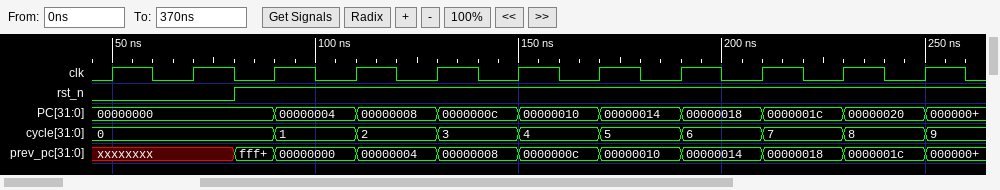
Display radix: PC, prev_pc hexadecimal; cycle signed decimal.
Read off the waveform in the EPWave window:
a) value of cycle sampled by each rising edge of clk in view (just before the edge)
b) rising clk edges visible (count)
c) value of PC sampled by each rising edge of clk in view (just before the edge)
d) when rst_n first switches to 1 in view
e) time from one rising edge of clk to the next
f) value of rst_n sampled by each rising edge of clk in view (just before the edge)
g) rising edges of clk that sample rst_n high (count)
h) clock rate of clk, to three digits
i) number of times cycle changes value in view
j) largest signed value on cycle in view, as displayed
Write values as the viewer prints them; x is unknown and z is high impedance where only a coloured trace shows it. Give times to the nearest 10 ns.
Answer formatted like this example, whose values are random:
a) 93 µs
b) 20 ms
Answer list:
a) 0, 0, 0, 1, 2, 3, 4, 5, 6, 7, 8
b) 11
c) 00000000, 00000000, 00000000, 00000004, 00000008, 0000000c, 00000010, 00000014, 00000018, 0000001c, 00000020
d) 80 ns
e) 20 ns
f) 0 0 1 1 1 1 1 1 1 1 1
g) 9
h) 50.0 MHz
i) 9
j) 9
